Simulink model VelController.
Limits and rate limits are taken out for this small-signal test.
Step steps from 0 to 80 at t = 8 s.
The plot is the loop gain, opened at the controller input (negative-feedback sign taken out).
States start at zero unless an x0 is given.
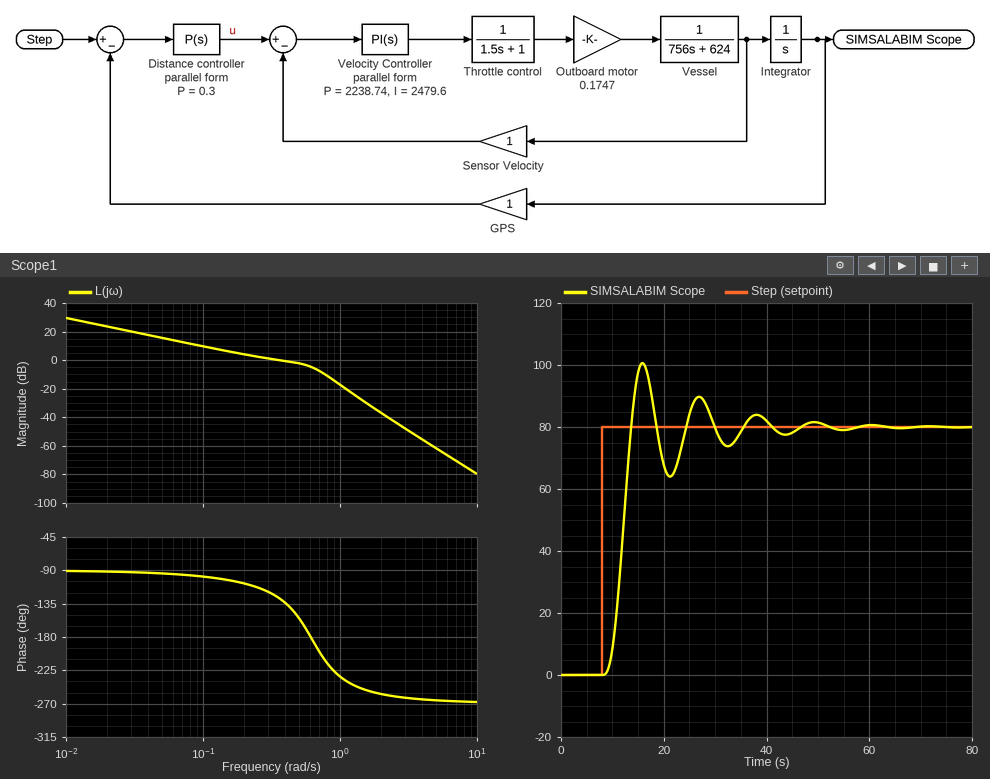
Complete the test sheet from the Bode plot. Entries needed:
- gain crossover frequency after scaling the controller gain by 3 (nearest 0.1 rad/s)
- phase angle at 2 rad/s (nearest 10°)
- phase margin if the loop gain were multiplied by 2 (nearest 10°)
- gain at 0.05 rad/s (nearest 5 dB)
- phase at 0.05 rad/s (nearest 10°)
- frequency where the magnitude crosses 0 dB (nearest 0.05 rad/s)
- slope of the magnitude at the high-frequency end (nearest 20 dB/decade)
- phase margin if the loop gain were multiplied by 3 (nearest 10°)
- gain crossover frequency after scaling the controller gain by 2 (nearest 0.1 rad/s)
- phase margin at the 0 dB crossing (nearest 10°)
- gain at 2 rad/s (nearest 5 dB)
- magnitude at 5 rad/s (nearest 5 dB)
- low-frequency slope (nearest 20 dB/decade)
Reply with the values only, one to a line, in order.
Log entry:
0.8 rad/s
-260°
-10°
15 dB
-90°
0.35 rad/s
-60 dB/decade
-30°
0.7 rad/s
50°
-35 dB
-60 dB
-20 dB/decade
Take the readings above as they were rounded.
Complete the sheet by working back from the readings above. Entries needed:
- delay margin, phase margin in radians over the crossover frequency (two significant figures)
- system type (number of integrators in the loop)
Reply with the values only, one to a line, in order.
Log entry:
2.5 s
1
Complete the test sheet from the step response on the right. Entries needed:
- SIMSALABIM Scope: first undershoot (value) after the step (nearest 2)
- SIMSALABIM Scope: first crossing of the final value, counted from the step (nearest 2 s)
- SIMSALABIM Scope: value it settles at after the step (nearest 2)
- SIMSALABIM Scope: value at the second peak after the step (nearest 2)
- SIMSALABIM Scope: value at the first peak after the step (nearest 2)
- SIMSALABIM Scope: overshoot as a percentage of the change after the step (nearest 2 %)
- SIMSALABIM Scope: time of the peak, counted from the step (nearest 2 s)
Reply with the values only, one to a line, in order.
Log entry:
64
6 s
80
90
100
26 %
8 s
